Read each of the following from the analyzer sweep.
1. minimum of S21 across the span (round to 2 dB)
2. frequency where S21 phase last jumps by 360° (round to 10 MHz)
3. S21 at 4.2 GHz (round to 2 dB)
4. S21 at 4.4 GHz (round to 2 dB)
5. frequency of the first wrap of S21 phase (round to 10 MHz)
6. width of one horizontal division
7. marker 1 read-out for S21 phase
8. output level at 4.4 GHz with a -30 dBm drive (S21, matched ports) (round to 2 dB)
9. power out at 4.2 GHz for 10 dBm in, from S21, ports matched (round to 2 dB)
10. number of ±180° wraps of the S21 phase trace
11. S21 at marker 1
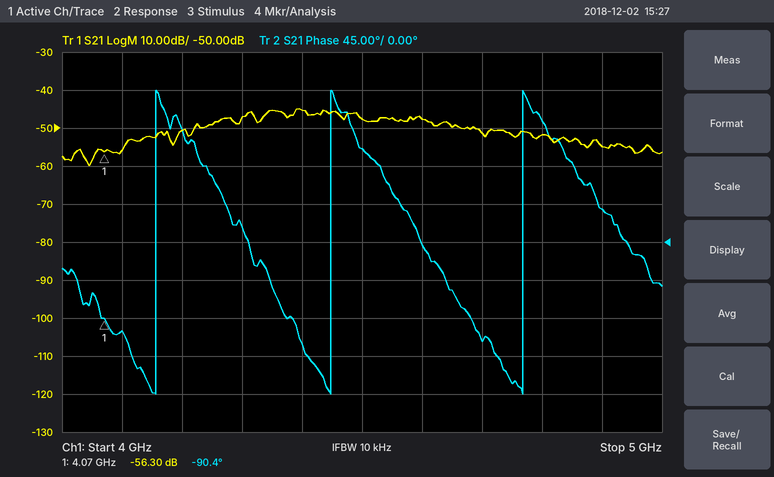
-60 dB
4.77 GHz
-50 dB
-46 dB
4.16 GHz
100 MHz
-90.4°
-76 dBm
-40 dBm
3
-56.30 dB
